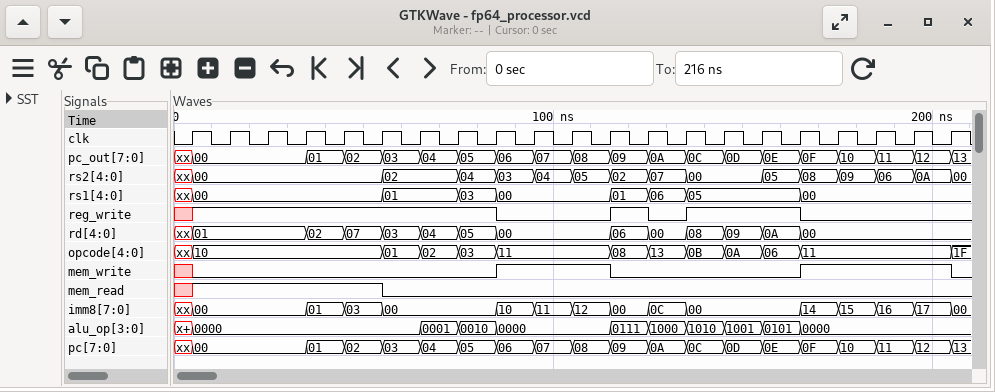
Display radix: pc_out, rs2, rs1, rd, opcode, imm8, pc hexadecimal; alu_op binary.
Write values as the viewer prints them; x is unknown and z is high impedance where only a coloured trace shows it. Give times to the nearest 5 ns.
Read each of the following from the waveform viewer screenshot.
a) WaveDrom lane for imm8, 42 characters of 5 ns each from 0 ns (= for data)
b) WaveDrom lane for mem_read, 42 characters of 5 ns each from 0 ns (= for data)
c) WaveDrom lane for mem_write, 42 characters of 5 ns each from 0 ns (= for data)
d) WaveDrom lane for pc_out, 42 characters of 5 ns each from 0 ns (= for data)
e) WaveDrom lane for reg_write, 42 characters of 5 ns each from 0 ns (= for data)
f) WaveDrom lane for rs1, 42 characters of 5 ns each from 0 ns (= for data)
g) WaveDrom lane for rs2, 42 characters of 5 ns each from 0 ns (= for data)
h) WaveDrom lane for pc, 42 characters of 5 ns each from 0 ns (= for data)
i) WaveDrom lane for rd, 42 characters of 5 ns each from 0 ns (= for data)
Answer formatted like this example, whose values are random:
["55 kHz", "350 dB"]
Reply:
["{name: 'imm8', wave: 'x=.....=.=.=.....=.=.=.=.=.=.....=.=.=.=.=', data: '00 01 03 00 10 11 12 00 0C 00 14 15 16 17 00'}", "{name: 'mem_read', wave: 'x1.........0..............................'}", "{name: 'mem_write', wave: 'x0...............1.....0.........1.......0'}", "{name: 'pc_out', wave: 'x=.....=.=.=.=.=.=.=.=.=.=.=.=.=.=.=.=.=.=', data: '00 01 02 03 04 05 06 07 08 09 0A 0C 0D 0E 0F 10 11 12 13'}", "{name: 'reg_write', wave: 'x1...............0.....1.0.1.....0........'}", "{name: 'rs1', wave: 'x=.........=...=.=.....=.=.=.....=........', data: '00 01 03 00 01 06 05 00'}", "{name: 'rs2', wave: 'x=.........=...=.=.=.=.=.=.=...=.=.=.=.=.=', data: '00 02 04 03 04 05 02 07 00 05 08 09 06 0A 00'}", "{name: 'pc', wave: 'x=.....=.=.=.=.=.=.=.=.=.=.=.=.=.=.=.=.=.=', data: '00 01 02 03 04 05 06 07 08 09 0A 0C 0D 0E 0F 10 11 12 13'}", "{name: 'rd', wave: 'x=.....=.=.=.=.=.=.....=.=.=.=.=.=........', data: '01 02 07 03 04 05 00 06 00 08 09 0A 00'}"]
